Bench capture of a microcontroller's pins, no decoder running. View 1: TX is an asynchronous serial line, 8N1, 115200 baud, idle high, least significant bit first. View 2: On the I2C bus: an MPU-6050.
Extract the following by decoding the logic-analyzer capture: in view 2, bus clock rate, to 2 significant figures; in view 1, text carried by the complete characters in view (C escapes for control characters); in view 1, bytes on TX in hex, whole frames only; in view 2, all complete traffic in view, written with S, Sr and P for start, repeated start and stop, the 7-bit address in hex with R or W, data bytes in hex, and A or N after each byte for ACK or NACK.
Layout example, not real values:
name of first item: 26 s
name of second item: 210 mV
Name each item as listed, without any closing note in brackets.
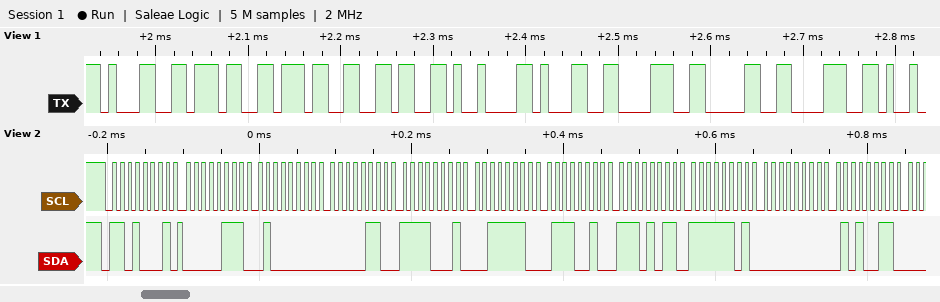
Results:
in view 2, bus clock rate, to 2 significant figures: 100 kHz
in view 1, text carried by the complete characters in view: "1776\t1808"
in view 1, bytes on TX in hex, whole frames only: 31 37 37 36 09 31 38 30 38
in view 2, all complete traffic in view, written with S, Sr and P for start, repeated start and stop, the 7-bit address in hex with R or W, data bytes in hex, and A or N after each byte for ACK or NACK: S 68R A 07 A 40 A 06 A F1 A 3E A 72 A EB A FD A 00 A 53 A
